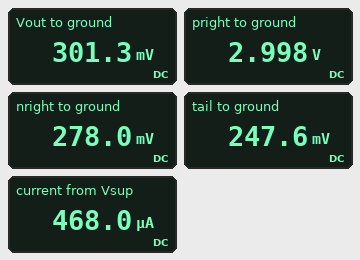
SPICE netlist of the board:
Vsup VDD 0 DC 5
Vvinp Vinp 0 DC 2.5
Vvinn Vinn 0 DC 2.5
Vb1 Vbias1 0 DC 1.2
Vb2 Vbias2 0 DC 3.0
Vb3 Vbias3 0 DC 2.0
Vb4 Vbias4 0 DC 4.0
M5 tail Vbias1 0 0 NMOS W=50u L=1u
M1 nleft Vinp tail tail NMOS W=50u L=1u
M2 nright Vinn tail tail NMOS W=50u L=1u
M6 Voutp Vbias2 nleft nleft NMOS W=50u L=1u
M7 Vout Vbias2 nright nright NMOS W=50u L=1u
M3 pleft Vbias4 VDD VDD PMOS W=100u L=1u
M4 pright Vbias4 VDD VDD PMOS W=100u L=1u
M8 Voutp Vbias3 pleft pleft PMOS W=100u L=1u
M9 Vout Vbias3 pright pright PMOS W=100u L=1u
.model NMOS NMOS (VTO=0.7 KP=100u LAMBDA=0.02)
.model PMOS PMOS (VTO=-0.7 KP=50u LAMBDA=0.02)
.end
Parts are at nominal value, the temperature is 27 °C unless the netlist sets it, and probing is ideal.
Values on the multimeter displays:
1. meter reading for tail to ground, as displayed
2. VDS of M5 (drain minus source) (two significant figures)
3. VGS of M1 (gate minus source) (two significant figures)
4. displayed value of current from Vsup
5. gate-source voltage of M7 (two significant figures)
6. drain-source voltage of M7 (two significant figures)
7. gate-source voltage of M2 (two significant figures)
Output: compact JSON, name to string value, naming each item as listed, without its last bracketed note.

{"meter reading for tail to ground, as displayed": "247.6 mV", "VDS of M5 (drain minus source)": "250 mV", "VGS of M1 (gate minus source)": "2.3 V", "displayed value of current from Vsup": "468.0 µA", "gate-source voltage of M7": "2.7 V", "drain-source voltage of M7": "23 mV", "gate-source voltage of M2": "2.3 V"}
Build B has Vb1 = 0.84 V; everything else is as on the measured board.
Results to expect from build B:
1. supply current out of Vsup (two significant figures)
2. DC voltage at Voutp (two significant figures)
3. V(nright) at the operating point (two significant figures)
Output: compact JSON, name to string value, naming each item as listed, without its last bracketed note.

{"supply current out of Vsup": "51 µA", "DC voltage at Voutp": "5.0 V", "V(nright) at the operating point": "2.2 V"}
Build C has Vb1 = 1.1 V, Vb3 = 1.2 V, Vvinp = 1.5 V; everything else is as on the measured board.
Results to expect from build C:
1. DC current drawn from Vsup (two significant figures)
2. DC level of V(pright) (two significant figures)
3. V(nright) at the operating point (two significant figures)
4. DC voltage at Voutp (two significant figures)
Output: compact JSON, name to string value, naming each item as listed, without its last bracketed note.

{"DC current drawn from Vsup": "400 µA", "DC level of V(pright)": "2.2 V", "V(nright) at the operating point": "580 mV", "DC voltage at Voutp": "4.8 V"}
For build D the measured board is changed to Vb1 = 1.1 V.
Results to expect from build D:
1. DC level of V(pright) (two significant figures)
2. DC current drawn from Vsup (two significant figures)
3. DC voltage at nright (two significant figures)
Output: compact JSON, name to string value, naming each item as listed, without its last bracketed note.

{"DC level of V(pright)": "4.8 V", "DC current drawn from Vsup": "410 µA", "DC voltage at nright": "2.0 V"}
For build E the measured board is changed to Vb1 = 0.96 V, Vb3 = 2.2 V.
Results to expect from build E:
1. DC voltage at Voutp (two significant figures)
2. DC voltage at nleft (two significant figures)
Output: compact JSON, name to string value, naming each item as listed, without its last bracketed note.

{"DC voltage at Voutp": "4.9 V", "DC voltage at nleft": "2.1 V"}
